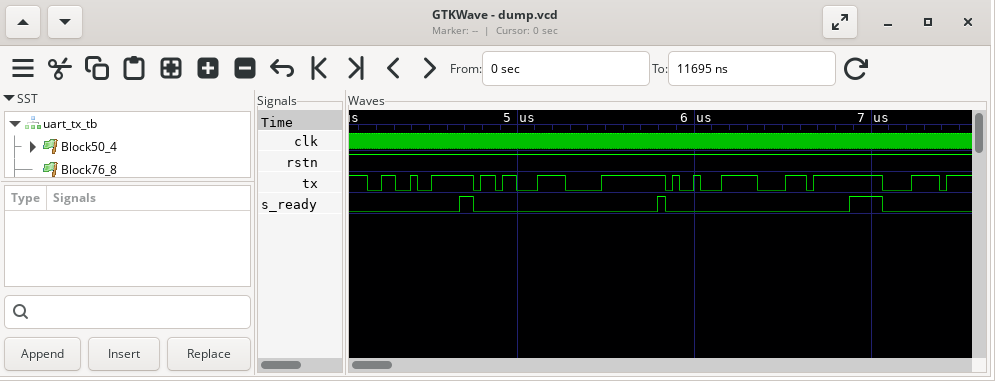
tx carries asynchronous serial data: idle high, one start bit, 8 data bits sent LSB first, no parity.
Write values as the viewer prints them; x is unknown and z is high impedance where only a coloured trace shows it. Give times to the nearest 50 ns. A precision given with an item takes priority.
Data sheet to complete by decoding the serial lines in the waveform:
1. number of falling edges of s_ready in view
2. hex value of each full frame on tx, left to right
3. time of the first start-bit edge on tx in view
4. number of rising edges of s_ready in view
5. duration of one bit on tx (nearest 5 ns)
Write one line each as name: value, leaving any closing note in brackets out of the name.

number of falling edges of s_ready in view: 3
hex value of each full frame on tx, left to right: 26, 1B, F0, 89, B8, 78
time of the first start-bit edge on tx in view: 4150 ns
number of rising edges of s_ready in view: 3
duration of one bit on tx: 40 ns
